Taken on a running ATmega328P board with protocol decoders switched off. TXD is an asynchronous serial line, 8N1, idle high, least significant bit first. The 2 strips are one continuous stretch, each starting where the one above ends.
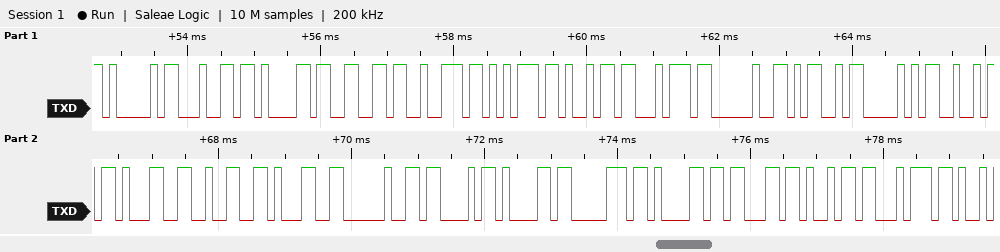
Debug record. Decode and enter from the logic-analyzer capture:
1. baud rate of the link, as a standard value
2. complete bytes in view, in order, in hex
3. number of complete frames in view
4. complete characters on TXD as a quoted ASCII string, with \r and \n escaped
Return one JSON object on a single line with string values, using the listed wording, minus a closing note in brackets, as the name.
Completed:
{"baud rate of the link, as a standard value": "9600 baud", "complete bytes in view, in order, in hex": "0x41 0x64 0x61 0x66 0x72 0x75 0x69 0x74 0x20 0x4D 0x50 0x52 0x31 0x32 0x31 0x20 0x43 0x61 0x70 0x61 0x63 0x69 0x74", "number of complete frames in view": "23", "complete characters on TXD as a quoted ASCII string, with \\r and \\n escaped": "\"Adafruit MPR121 Capacit\""}
